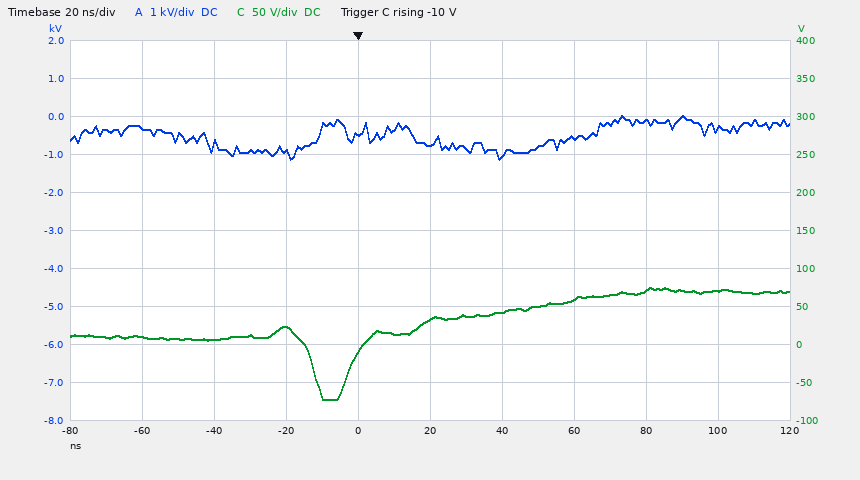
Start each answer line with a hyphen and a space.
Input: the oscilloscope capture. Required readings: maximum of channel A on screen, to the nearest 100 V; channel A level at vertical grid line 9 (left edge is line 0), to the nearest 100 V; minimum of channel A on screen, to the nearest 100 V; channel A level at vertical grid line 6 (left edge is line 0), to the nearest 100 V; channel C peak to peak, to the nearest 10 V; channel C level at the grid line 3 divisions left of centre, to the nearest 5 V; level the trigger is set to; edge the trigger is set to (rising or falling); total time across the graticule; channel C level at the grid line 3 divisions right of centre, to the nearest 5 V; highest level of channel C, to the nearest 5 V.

- 0.0 kV
- -300 V
- -1.1 kV
- -1.0 kV
- 150 V
- 5 V
- -10 V
- rising
- 200 ns
- 70 V
- 75 V
